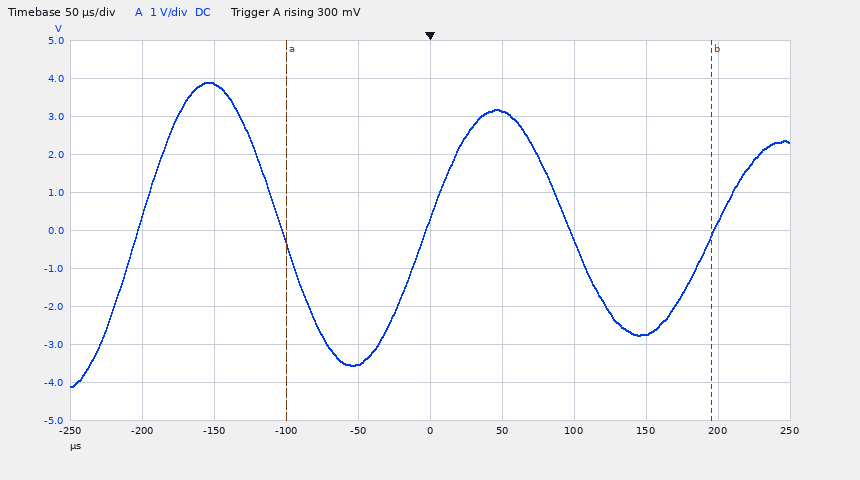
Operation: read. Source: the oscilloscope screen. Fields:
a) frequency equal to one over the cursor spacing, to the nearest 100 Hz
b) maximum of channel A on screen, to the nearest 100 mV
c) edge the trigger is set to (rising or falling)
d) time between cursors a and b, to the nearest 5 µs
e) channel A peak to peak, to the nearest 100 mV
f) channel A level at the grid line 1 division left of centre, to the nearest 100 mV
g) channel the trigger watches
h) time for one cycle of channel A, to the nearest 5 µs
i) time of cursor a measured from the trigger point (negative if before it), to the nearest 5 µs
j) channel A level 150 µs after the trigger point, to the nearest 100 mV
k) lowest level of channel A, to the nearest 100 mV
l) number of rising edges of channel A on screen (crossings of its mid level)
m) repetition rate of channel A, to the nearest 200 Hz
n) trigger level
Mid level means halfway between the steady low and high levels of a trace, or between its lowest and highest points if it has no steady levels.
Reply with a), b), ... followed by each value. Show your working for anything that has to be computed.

a) 1 / 295 µs ≈ 3.4 kHz
b) 3.9 V
c) rising
d) 295 µs
e) 3.9 V − (-4.1 V) = 8.0 V
f) -3.5 V
g) channel A
h) 200 µs
i) -100 µs
j) -2.7 V
k) -4.1 V
l) 3
m) 1 / 200 µs ≈ 5.0 kHz
n) 300 mV
